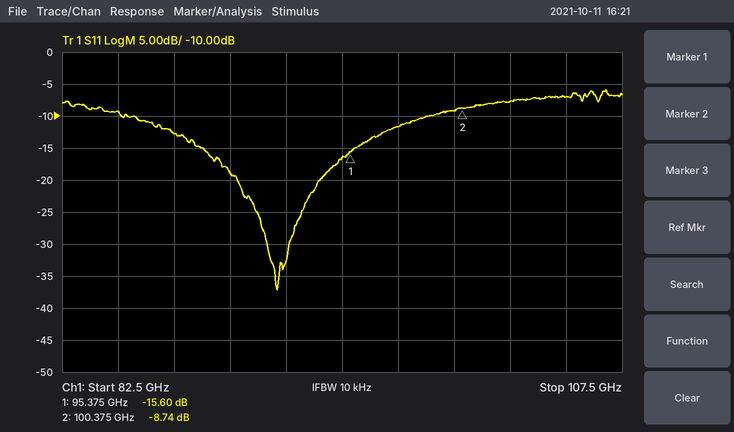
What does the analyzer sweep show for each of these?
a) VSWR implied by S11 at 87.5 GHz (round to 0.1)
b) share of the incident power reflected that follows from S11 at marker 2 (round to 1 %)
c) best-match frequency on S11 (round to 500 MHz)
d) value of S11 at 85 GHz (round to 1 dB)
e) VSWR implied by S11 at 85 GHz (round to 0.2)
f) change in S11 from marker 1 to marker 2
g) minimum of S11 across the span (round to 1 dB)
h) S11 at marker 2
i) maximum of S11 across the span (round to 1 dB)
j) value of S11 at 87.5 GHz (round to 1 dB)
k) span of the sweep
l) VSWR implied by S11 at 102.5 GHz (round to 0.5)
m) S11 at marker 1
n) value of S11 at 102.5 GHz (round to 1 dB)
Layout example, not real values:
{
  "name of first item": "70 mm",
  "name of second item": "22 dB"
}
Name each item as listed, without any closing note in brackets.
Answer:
{
  "VSWR implied by S11 at 87.5 GHz": "1.6",
  "share of the incident power reflected that follows from S11 at marker 2": "13 %",
  "best-match frequency on S11": "92.0 GHz",
  "value of S11 at 85 GHz": "-9 dB",
  "VSWR implied by S11 at 85 GHz": "2.0",
  "change in S11 from marker 1 to marker 2": "6.86 dB",
  "minimum of S11 across the span": "-37 dB",
  "S11 at marker 2": "-8.74 dB",
  "maximum of S11 across the span": "-6 dB",
  "value of S11 at 87.5 GHz": "-13 dB",
  "span of the sweep": "25 GHz",
  "VSWR implied by S11 at 102.5 GHz": "2.5",
  "S11 at marker 1": "-15.60 dB",
  "value of S11 at 102.5 GHz": "-8 dB"
}
